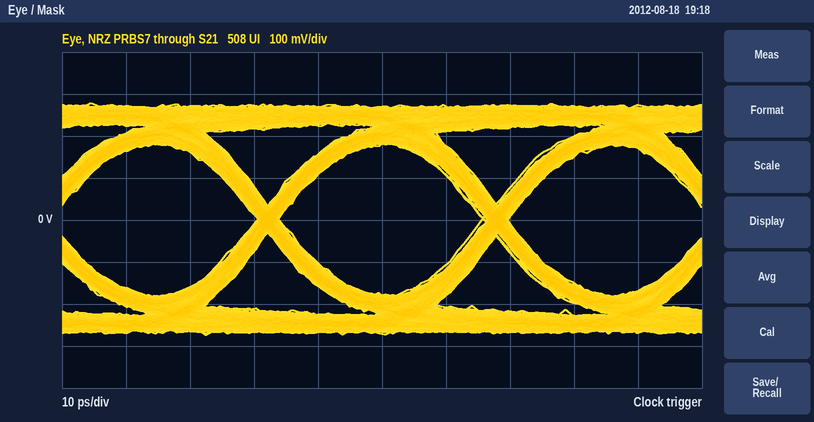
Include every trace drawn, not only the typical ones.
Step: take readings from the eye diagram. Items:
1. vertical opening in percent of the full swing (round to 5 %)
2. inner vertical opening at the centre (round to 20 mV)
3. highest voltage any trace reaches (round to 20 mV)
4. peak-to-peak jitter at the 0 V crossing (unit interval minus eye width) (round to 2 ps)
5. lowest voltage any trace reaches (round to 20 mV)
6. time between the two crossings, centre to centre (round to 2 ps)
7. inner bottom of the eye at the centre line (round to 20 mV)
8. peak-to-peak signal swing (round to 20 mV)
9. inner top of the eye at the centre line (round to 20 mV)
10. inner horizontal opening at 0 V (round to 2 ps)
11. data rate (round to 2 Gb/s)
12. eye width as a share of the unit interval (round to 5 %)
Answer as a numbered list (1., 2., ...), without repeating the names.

1. 65 %
2. 360 mV
3. 280 mV
4. 4 ps
5. -280 mV
6. 36 ps
7. -180 mV
8. 560 mV
9. 180 mV
10. 32 ps
11. 28 Gb/s
12. 90 %
